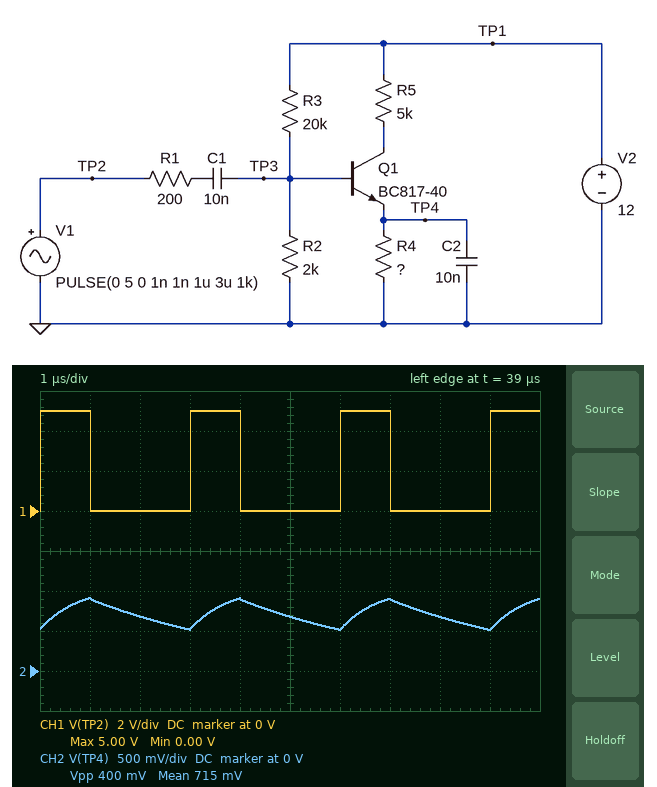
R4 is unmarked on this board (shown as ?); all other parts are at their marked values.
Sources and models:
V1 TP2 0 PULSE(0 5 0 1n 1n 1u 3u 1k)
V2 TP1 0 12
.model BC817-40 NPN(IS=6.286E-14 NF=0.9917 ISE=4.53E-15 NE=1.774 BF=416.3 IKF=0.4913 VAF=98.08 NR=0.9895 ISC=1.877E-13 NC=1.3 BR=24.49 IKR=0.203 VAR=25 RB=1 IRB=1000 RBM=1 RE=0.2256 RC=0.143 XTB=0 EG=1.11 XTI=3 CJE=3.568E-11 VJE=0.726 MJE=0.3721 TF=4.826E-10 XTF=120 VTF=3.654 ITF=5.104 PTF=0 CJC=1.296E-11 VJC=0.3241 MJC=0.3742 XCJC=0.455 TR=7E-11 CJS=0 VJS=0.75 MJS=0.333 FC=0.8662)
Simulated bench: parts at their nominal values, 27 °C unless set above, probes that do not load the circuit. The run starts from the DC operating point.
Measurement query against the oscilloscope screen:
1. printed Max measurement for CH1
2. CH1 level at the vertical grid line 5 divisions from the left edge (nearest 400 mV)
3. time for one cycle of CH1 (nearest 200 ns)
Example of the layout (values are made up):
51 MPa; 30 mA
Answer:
5.00 V; 0 V; 3.0 µs
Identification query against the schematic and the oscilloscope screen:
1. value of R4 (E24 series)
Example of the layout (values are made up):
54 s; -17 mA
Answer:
360 Ω
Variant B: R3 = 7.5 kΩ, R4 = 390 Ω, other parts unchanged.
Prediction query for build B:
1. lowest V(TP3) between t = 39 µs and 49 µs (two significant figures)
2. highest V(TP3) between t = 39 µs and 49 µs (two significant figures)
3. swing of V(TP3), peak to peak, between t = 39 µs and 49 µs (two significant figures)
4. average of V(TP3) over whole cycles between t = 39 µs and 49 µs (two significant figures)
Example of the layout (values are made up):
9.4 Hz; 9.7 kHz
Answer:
-1.7 V; 2.0 V; 3.8 V; -400 mV
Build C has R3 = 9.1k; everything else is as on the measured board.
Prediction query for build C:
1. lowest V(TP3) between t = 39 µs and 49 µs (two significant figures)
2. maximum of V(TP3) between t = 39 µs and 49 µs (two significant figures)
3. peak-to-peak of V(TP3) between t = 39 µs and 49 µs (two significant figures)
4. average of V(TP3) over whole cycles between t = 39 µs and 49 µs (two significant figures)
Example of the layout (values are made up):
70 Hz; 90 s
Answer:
-2.0 V; 1.9 V; 3.8 V; -610 mV
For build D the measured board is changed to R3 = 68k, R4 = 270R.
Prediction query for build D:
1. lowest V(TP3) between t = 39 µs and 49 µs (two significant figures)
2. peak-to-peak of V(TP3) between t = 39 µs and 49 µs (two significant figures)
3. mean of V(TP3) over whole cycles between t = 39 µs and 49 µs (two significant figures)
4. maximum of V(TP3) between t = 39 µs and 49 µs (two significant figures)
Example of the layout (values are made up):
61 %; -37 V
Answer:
-2.9 V; 4.2 V; -1.4 V; 1.3 V
